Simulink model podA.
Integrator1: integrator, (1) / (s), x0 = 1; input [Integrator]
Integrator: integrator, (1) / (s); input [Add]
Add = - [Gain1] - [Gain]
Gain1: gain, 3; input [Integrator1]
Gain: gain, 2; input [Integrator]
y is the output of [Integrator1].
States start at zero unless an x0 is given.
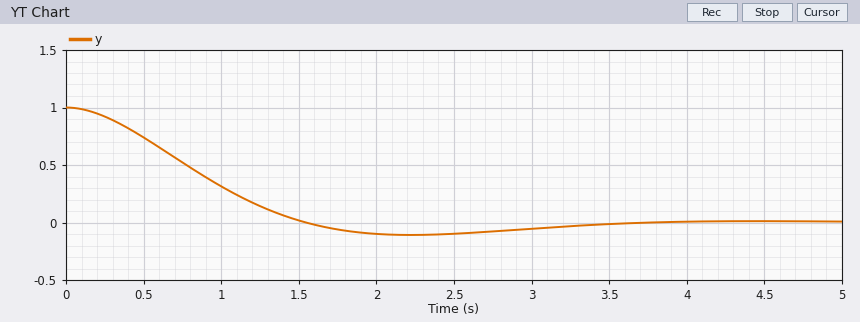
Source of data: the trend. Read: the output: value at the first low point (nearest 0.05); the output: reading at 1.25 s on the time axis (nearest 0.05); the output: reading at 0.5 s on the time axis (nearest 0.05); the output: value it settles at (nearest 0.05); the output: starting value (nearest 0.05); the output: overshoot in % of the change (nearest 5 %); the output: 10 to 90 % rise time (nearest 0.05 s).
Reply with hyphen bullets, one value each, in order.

- -0.10
- 0.15
- 0.75
- 0.00
- 1.00
- 10 %
- 1.05 s
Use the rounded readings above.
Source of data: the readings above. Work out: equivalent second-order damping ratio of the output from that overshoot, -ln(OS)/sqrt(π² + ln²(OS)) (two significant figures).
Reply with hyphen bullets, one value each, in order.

- 0.59
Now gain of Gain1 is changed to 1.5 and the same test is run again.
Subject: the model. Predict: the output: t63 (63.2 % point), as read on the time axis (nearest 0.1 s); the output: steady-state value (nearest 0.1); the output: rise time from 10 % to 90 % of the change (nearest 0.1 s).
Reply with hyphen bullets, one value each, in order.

- 1.5 s
- 0.0
- 2.1 s
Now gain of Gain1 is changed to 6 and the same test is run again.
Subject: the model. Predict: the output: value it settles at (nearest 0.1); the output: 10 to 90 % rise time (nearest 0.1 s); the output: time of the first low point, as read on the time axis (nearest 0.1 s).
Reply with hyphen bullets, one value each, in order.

- 0.0
- 0.6 s
- 1.4 s
